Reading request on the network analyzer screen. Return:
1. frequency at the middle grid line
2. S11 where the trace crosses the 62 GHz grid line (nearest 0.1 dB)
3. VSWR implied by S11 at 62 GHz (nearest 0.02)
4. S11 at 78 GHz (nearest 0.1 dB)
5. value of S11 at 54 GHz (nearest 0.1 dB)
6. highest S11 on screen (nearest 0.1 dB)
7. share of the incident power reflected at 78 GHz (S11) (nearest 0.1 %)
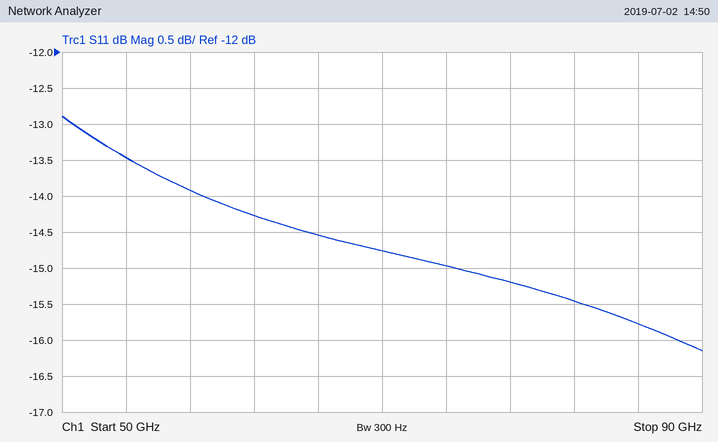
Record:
70 GHz
-14.3 dB
1.48
-15.2 dB
-13.5 dB
-12.9 dB
3.0 %
